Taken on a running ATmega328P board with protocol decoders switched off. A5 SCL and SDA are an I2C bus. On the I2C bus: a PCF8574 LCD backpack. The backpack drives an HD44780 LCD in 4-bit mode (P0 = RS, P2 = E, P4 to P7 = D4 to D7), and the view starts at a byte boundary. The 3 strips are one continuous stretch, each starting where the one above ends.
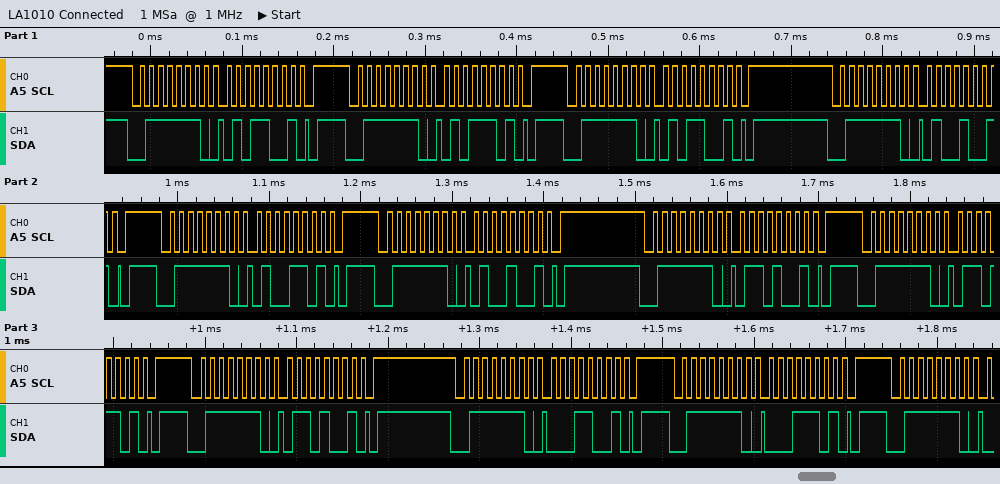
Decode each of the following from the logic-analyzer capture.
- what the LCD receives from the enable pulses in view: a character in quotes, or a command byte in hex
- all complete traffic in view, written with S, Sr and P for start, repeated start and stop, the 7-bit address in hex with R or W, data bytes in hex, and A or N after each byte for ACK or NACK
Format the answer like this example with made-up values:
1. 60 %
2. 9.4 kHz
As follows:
1. 'T'
2. S 3FW A 59 A P S 3FW A 5D A P S 3FW A 59 A P S 3FW A 49 A P S 3FW A 4D A P S 3FW A 49 A P S 3FW A 69 A P S 3FW A 6D A P S 3FW A 69 A P S 3FW A 19 A P S 3FW A 1D A P S 3FW A
